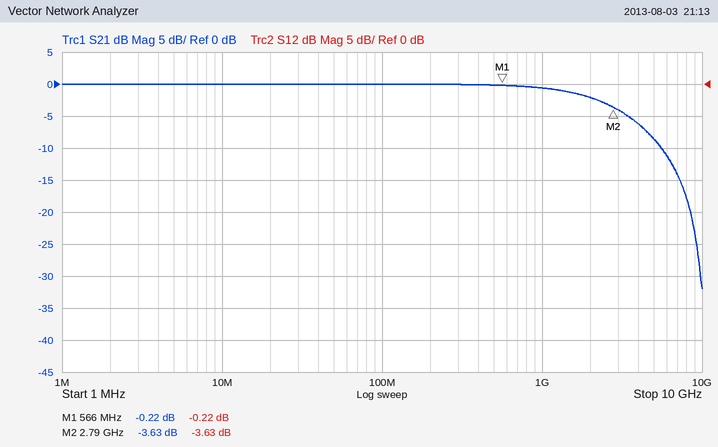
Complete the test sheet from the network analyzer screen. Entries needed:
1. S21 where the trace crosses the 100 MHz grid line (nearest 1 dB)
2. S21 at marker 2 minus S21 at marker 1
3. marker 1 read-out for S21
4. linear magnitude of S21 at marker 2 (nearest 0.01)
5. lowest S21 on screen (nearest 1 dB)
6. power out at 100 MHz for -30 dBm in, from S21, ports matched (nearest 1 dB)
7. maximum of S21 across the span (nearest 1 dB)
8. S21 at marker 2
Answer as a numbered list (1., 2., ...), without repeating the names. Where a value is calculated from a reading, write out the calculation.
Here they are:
1. 0 dB
2. -3.63 − (-0.22) = -3.41 dB
3. -0.22 dB
4. 10^(-3.63/20) ≈ 0.66
5. -32 dB
6. -30 dBm + (0 dB) = -30 dBm
7. 0 dB
8. -3.63 dB
